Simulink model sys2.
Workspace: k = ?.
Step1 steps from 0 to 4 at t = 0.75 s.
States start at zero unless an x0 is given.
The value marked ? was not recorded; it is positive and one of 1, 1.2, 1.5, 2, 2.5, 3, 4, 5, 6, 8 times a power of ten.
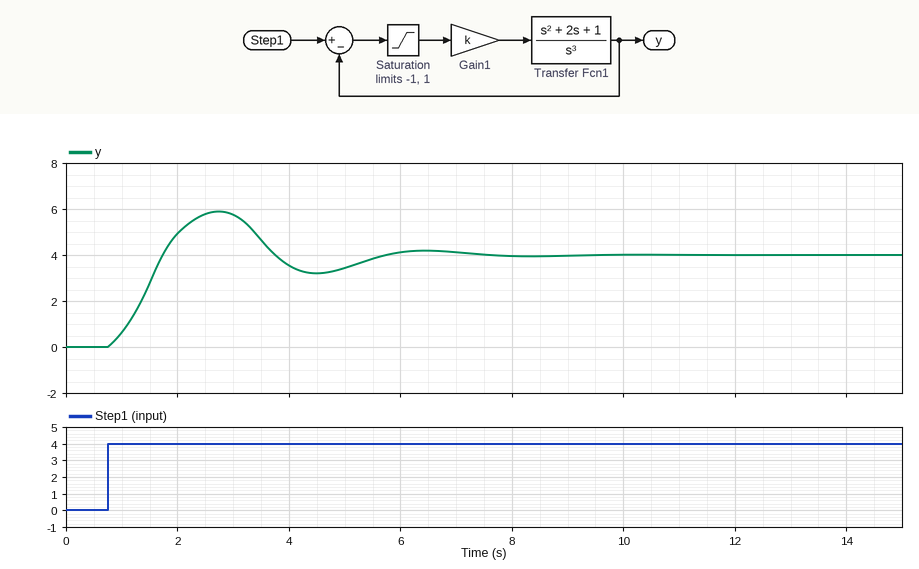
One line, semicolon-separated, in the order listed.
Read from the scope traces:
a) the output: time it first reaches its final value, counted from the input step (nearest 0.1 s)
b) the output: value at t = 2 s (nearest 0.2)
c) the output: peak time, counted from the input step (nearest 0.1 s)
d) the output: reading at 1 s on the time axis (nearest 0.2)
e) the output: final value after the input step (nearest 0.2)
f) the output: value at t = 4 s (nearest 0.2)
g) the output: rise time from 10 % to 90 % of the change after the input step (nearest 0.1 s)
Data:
1.0 s; 5.0; 2.0 s; 0.6; 4.0; 3.6; 0.7 s
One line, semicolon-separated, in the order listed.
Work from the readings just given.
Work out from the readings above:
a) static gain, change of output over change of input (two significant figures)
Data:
1.0
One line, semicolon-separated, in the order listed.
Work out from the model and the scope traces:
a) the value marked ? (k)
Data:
2
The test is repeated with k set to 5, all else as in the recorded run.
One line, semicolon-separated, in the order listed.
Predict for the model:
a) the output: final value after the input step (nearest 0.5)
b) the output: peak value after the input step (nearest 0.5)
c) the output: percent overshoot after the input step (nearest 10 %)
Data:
4.0; 5.0; 20 %
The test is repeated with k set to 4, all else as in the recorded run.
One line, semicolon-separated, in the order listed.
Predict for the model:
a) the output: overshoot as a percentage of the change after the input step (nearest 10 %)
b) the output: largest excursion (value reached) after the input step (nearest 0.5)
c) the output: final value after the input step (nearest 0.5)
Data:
20 %; 5.0; 4.0
